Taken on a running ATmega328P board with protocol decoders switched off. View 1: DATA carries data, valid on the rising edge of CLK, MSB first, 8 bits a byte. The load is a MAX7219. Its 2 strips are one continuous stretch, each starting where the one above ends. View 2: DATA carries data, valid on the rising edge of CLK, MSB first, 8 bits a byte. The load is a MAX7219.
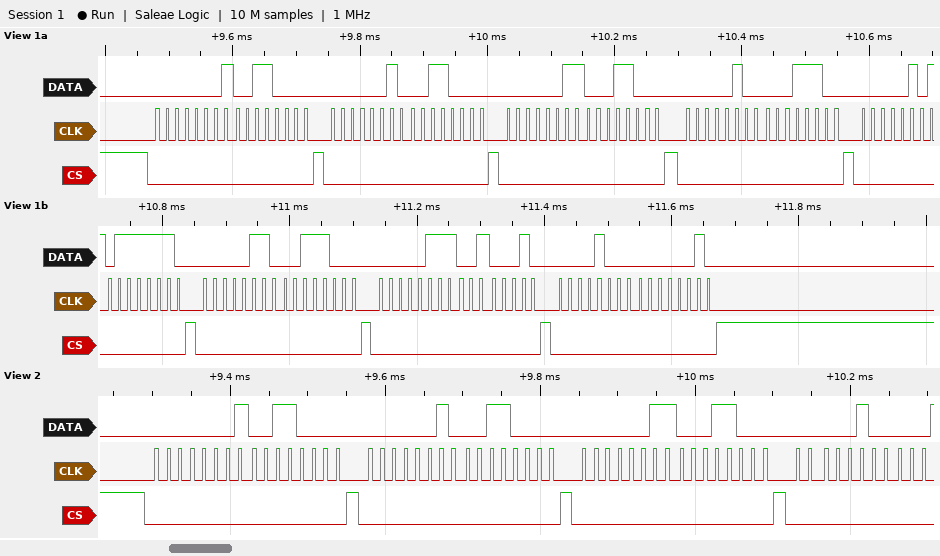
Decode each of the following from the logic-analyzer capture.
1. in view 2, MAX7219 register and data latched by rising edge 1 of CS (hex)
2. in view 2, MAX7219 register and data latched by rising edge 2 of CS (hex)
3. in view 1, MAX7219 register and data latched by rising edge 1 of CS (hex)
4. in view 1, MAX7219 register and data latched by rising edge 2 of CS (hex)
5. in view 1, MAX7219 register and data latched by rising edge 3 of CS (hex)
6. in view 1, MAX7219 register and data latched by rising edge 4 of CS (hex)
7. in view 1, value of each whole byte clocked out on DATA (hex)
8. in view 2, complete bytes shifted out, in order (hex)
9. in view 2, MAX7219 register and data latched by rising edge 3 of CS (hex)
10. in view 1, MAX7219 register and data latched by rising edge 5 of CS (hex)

register 0x1, data 0x30
register 0x2, data 0x30
register 0x1, data 0x30
register 0x2, data 0x30
register 0x3, data 0x18
register 0x4, data 0x1C
01 30 02 30 03 18 04 1C 05 7E 06 38 07 22 08 02
01 30 02 30 03 18 04
register 0x3, data 0x18
register 0x5, data 0x7E
